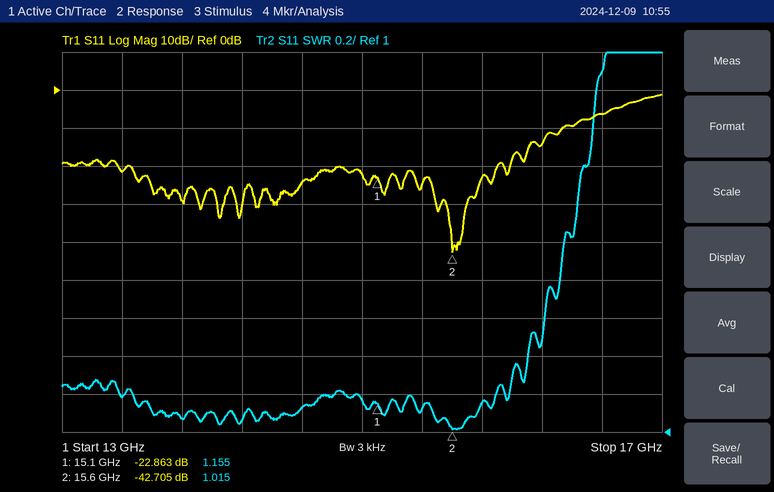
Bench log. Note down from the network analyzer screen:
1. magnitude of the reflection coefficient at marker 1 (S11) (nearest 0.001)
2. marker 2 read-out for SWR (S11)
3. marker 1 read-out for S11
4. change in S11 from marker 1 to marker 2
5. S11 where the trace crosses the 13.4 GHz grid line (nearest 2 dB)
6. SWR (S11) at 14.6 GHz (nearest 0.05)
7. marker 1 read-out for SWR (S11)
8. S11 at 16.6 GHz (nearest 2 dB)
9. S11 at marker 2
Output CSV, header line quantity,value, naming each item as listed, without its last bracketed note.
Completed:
quantity,value
magnitude of the reflection coefficient at marker 1 (S11),0.072
marker 2 read-out for SWR,1.015
marker 1 read-out for S11,-22.863 dB
change in S11 from marker 1 to marker 2,-19.842 dB
S11 where the trace crosses the 13.4 GHz grid line,-22 dB
SWR (S11) at 14.6 GHz,1.15
marker 1 read-out for SWR,1.155
S11 at 16.6 GHz,-6 dB
S11 at marker 2,-42.705 dB
